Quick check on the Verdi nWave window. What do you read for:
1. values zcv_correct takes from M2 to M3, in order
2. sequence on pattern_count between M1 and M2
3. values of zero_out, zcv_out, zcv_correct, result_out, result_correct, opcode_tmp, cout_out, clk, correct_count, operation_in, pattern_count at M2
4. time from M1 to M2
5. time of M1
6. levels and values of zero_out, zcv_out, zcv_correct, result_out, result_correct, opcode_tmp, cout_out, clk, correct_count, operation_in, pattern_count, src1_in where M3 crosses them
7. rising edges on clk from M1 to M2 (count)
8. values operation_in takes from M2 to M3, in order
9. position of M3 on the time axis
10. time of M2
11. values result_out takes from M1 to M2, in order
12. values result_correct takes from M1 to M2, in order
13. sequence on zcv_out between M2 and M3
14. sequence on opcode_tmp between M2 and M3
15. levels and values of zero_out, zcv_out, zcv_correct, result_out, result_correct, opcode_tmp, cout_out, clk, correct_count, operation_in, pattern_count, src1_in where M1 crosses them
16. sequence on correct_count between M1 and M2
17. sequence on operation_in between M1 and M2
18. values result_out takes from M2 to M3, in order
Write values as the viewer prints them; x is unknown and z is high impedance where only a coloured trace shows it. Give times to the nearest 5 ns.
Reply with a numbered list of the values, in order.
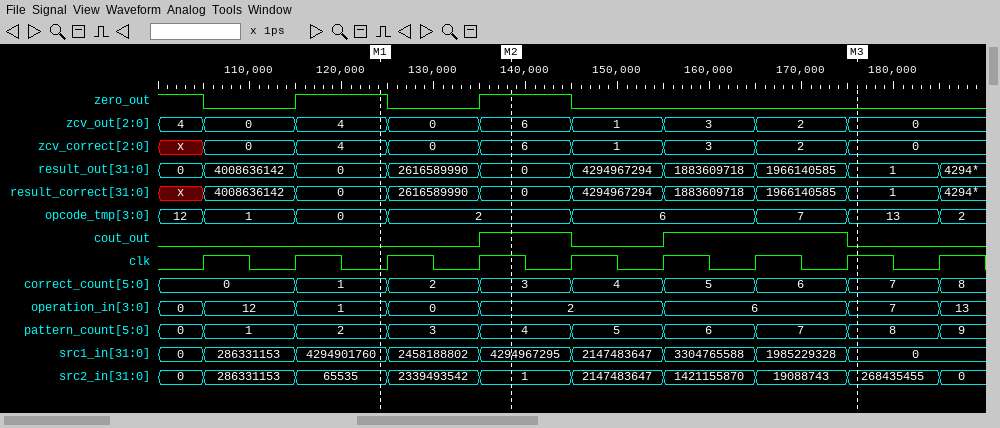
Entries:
1. 6, 1, 3, 2, 0
2. 2, 3, 4
3. zero_out=1, zcv_out=6, zcv_correct=6, result_out=0, result_correct=0, opcode_tmp=2, cout_out=1, clk=1, correct_count=3, operation_in=2, pattern_count=4
4. 15 ns
5. 125 ns
6. zero_out=0, zcv_out=0, zcv_correct=0, result_out=1, result_correct=1, opcode_tmp=13, cout_out=0, clk=1, correct_count=7, operation_in=7, pattern_count=8, src1_in=0
7. 2
8. 2, 6, 7
9. 175 ns
10. 140 ns
11. 0, 2616589990, 0
12. 0, 2616589990, 0
13. 6, 1, 3, 2, 0
14. 2, 6, 7, 13
15. zero_out=1, zcv_out=4, zcv_correct=4, result_out=0, result_correct=0, opcode_tmp=0, cout_out=0, clk=0, correct_count=1, operation_in=1, pattern_count=2, src1_in=4294901760
16. 1, 2, 3
17. 1, 0, 2
18. 0, 4294967294, 1883609718, 1966140585, 1
